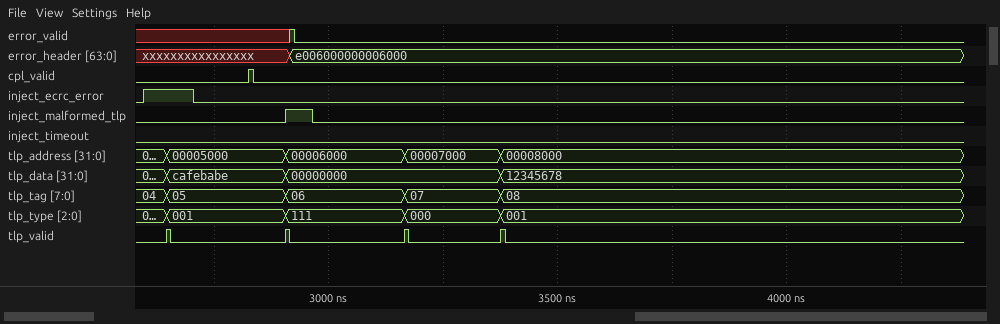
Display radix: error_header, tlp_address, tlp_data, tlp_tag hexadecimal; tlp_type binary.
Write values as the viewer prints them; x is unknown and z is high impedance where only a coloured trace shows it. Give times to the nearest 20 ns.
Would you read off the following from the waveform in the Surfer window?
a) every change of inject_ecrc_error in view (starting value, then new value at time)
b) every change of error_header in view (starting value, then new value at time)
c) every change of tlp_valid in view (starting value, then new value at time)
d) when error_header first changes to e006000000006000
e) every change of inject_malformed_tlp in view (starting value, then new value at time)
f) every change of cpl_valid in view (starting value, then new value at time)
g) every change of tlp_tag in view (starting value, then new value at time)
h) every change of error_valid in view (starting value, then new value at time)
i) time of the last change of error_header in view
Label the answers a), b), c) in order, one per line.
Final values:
a) 0, 1 at 2600 ns, 0 at 2700 ns
b) xxxxxxxxxxxxxxxx, e006000000006000 at 2920 ns
c) 0, 1 at 2640 ns, 0 at 2660 ns, 1 at 2900 ns, 0 at 2920 ns, 1 at 3160 ns, 0 at 3180 ns, 1 at 3380 ns, 0 at 3380 ns
d) 2920 ns
e) 0, 1 at 2900 ns, 0 at 2960 ns
f) 0, 1 at 2820 ns, 0 at 2840 ns
g) 04, 05 at 2640 ns, 06 at 2900 ns, 07 at 3160 ns, 08 at 3380 ns
h) x, 1 at 2920 ns, 0 at 2920 ns
i) 2920 ns
